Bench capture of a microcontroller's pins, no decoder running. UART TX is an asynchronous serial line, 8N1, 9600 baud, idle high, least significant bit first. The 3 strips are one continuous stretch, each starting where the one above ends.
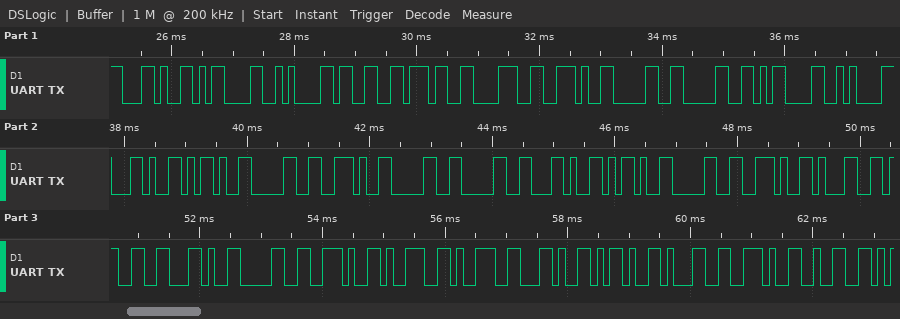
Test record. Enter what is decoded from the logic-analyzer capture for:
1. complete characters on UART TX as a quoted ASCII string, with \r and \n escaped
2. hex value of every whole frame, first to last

",\r\n378.00\r\n,-0.00,-0.13,0.99,-1.2"
0x2C 0x0D 0x0A 0x33 0x37 0x38 0x2E 0x30 0x30 0x0D 0x0A 0x2C 0x2D 0x30 0x2E 0x30 0x30 0x2C 0x2D 0x30 0x2E 0x31 0x33 0x2C 0x30 0x2E 0x39 0x39 0x2C 0x2D 0x31 0x2E 0x32
